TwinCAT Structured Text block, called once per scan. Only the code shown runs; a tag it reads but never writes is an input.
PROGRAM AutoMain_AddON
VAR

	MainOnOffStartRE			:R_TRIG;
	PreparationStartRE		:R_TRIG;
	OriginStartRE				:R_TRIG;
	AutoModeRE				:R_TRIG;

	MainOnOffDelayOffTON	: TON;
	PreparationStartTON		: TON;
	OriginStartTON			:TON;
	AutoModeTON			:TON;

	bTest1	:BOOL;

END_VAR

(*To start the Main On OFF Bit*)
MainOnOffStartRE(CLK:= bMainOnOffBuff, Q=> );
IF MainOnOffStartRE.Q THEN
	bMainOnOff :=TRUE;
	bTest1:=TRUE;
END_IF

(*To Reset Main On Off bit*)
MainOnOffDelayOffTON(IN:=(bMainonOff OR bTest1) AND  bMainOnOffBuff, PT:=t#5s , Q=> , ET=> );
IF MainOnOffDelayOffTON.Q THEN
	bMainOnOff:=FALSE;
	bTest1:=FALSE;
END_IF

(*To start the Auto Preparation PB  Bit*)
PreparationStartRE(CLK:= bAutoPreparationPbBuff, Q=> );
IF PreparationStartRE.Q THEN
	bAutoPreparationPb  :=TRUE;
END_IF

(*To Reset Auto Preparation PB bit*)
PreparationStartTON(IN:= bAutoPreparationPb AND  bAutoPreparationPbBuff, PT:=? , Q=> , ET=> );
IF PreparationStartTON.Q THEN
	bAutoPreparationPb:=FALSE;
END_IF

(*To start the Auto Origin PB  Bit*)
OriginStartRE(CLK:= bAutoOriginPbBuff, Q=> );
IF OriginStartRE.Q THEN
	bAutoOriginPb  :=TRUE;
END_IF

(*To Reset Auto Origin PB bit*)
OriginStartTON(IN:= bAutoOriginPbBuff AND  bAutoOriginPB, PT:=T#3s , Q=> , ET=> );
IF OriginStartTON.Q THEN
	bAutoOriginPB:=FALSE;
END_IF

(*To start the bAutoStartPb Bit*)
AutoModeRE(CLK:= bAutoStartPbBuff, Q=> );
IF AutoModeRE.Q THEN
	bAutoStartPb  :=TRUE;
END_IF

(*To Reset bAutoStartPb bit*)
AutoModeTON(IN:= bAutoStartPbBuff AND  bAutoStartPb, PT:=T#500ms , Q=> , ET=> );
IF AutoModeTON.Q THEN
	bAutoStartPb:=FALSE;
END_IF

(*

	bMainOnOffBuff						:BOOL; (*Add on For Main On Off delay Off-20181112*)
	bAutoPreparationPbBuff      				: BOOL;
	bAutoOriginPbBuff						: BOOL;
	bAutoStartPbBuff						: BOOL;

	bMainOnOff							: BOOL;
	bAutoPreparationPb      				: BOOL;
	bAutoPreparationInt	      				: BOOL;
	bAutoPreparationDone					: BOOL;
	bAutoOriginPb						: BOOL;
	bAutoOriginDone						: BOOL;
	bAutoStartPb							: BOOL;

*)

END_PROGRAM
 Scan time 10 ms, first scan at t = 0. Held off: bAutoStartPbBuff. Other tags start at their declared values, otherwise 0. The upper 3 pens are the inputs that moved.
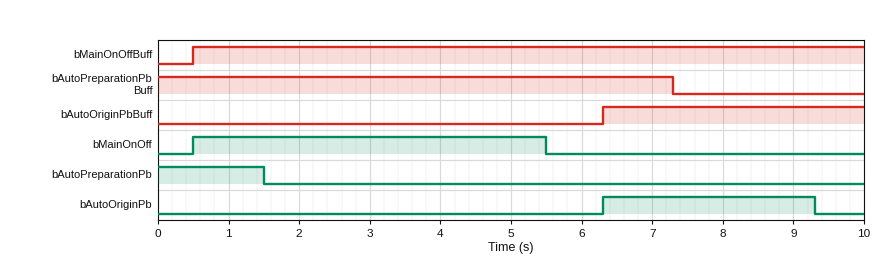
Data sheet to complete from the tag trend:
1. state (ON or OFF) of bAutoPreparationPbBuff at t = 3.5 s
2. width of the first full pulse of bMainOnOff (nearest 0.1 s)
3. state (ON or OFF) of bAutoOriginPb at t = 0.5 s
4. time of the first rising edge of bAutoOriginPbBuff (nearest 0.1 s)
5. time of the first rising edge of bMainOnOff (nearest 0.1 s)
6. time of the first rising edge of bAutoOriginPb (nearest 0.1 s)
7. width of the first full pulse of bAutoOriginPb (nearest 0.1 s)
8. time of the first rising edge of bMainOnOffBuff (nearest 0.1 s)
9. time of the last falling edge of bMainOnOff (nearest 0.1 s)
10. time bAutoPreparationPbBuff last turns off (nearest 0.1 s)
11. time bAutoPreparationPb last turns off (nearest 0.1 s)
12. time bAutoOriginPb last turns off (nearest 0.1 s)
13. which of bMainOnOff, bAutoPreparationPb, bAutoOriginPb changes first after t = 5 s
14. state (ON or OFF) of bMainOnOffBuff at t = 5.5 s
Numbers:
ON
5.0 s
OFF
6.3 s
0.5 s
6.3 s
3.0 s
0.5 s
5.5 s
7.3 s
1.5 s
9.3 s
bMainOnOff
ON
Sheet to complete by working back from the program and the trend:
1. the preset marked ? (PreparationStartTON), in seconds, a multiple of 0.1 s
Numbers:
1.5 s
